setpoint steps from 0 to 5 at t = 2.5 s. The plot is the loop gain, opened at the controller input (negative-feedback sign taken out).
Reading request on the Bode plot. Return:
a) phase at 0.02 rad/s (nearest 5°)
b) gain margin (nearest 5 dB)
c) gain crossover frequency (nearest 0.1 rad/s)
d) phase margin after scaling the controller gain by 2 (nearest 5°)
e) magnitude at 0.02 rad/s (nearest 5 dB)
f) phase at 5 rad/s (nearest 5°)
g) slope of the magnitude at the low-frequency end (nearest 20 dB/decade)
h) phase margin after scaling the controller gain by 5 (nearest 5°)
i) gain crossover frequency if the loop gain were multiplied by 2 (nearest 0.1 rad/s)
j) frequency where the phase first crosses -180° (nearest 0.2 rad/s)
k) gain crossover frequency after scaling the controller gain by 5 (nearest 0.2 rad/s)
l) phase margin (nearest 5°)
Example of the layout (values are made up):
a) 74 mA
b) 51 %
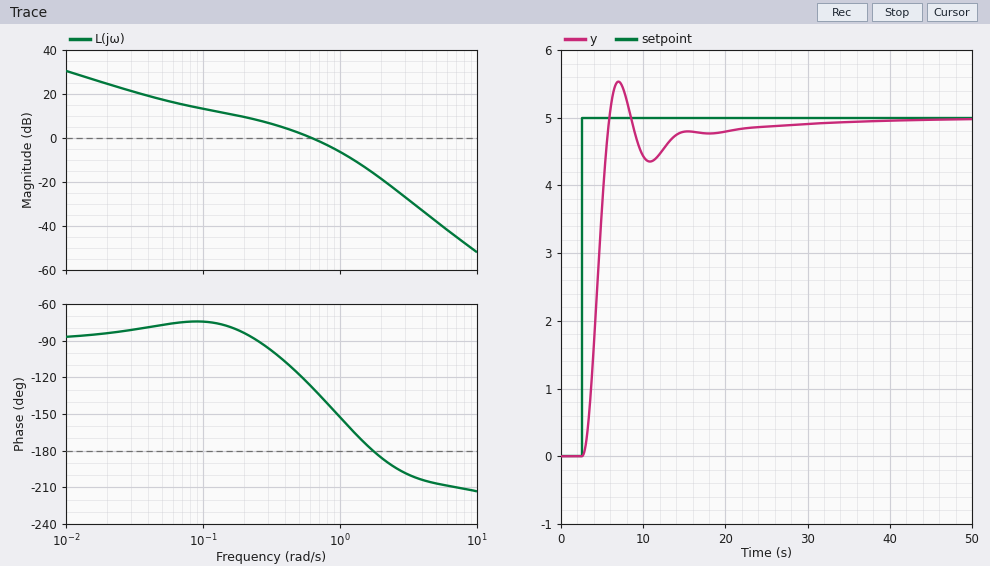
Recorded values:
a) -85°
b) 15 dB
c) 0.6 rad/s
d) 30°
e) 25 dB
f) -205°
g) -20 dB/decade
h) 5°
i) 1.0 rad/s
j) 1.8 rad/s
k) 1.6 rad/s
l) 50°
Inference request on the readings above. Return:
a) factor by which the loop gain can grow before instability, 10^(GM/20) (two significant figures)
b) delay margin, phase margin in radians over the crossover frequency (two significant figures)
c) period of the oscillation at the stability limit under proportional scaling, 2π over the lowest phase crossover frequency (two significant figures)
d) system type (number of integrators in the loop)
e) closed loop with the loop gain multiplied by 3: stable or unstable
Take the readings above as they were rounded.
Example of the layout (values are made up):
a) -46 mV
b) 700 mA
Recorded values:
a) 5.6
b) 1.5 s
c) 3.5 s
d) 1
e) stable
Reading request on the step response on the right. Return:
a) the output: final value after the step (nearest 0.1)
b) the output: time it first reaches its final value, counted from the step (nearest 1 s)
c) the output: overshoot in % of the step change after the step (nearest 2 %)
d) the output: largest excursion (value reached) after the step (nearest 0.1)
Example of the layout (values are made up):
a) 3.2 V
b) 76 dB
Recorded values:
a) 5.0
b) 3 s
c) 10 %
d) 5.5
